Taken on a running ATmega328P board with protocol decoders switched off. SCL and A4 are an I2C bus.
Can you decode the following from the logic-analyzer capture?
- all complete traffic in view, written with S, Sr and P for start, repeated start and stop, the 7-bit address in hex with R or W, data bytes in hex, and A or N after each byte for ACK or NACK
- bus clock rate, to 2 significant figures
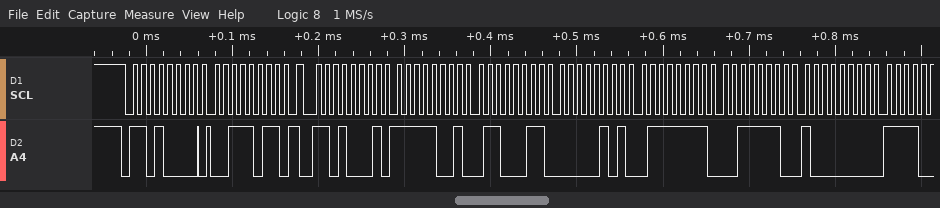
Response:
S 68W A 3B A Sr 68R A F9 A 63 A 05 A 7F A 3E A 80 A
100 kHz
